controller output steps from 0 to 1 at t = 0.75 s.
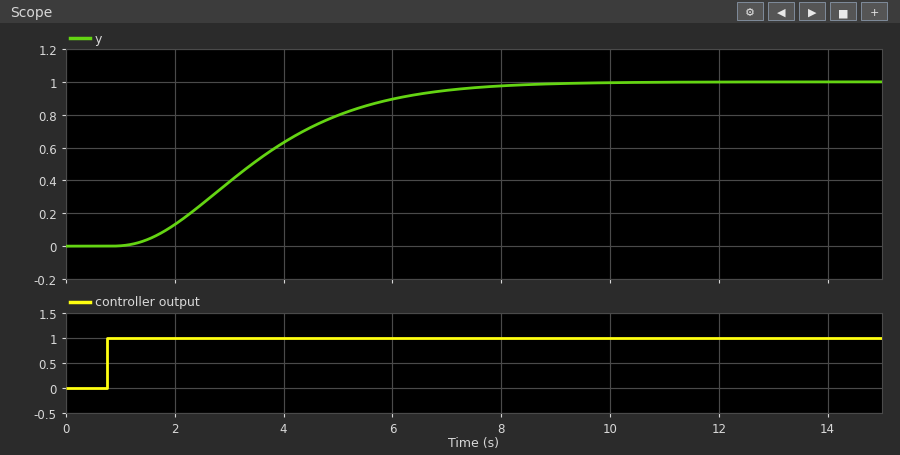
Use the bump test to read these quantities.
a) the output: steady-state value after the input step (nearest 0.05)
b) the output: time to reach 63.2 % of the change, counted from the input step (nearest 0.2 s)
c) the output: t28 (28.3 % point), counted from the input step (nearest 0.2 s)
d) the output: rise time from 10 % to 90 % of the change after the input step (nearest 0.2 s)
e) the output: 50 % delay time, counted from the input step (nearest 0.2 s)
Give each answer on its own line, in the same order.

1.00
3.2 s
1.8 s
4.2 s
2.6 s
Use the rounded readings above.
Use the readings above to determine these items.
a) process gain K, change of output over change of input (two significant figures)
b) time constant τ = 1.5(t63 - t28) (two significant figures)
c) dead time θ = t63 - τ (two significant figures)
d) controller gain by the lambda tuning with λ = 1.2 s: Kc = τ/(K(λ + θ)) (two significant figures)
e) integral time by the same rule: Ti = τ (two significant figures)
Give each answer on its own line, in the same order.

1.0
2.1 s
1.1 s
0.91
2.1 s
